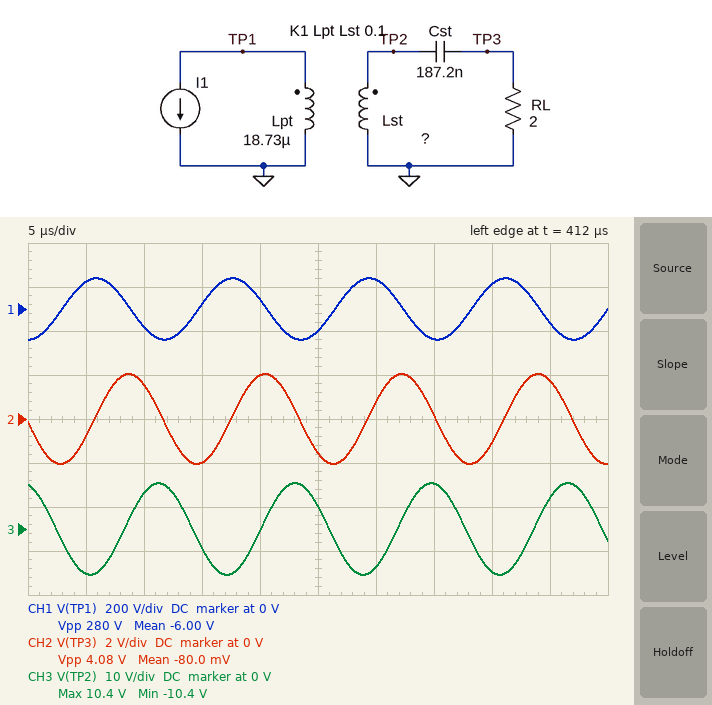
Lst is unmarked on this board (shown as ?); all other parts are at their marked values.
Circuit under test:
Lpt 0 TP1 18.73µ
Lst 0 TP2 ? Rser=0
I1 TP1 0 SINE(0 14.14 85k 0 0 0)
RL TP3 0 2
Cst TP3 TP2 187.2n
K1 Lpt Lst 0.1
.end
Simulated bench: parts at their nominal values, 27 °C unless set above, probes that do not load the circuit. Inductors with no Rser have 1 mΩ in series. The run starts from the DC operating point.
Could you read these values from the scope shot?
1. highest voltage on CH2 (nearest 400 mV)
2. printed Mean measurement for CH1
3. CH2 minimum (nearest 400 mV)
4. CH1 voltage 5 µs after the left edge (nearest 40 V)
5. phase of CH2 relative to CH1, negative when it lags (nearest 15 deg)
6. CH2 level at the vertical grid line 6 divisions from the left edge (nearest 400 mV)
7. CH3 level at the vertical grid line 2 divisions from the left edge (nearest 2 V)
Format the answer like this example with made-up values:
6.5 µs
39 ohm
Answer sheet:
2.0 V
-6.00 V
-2.0 V
120 V
-90 deg
800 mV
8 V
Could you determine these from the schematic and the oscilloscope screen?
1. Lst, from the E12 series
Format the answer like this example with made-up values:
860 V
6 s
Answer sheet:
68 µH
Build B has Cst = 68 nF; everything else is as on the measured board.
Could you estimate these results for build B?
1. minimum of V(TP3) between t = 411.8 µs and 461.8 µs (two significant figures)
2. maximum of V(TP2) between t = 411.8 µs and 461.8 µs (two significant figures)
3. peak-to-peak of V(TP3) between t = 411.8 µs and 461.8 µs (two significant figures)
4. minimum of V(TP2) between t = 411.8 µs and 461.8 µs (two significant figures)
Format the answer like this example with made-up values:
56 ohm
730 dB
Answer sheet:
-6.0 V
83 V
12 V
-83 V
